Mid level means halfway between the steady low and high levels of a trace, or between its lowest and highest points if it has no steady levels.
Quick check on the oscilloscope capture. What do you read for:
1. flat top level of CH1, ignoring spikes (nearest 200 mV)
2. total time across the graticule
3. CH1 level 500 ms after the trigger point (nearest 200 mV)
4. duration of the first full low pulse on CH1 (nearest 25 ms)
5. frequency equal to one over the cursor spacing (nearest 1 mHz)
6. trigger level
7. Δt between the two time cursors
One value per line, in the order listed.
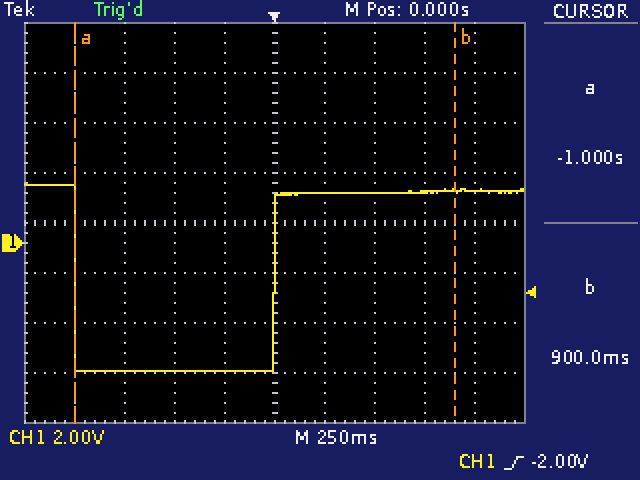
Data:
2.0 V
2.5 s
2.0 V
1.000 s
526 mHz
-2.00 V
1.900 s
